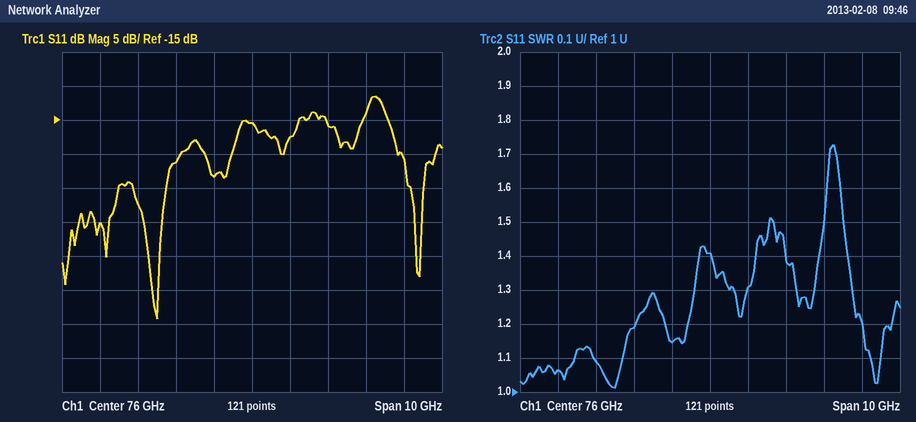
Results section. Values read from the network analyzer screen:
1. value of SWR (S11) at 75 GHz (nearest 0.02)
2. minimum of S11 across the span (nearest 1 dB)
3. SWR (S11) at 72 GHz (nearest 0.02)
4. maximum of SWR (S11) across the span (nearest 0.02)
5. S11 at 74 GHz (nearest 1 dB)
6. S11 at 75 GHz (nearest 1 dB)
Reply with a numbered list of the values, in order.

1. 1.14
2. -44 dB
3. 1.06
4. 1.72
5. -21 dB
6. -23 dB
